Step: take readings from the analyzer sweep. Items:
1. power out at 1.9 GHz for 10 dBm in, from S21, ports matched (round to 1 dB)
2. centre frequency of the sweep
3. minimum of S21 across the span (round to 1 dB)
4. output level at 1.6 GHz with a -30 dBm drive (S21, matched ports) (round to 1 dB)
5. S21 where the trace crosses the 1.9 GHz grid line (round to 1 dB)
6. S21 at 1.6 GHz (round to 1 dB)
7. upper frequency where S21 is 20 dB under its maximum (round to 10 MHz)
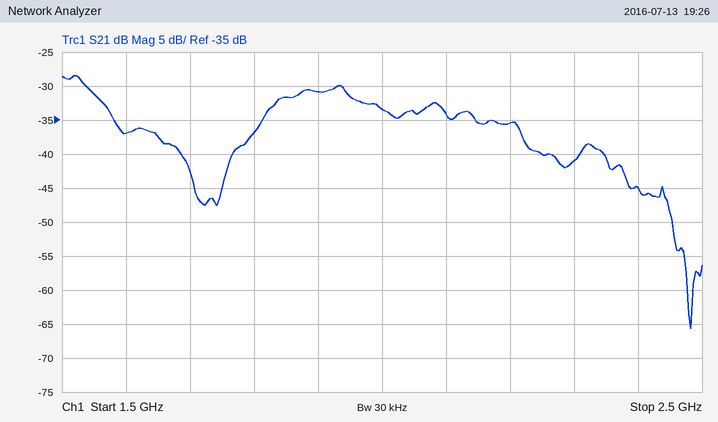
-21 dBm
2 GHz
-66 dB
-67 dBm
-31 dB
-37 dB
2.45 GHz
